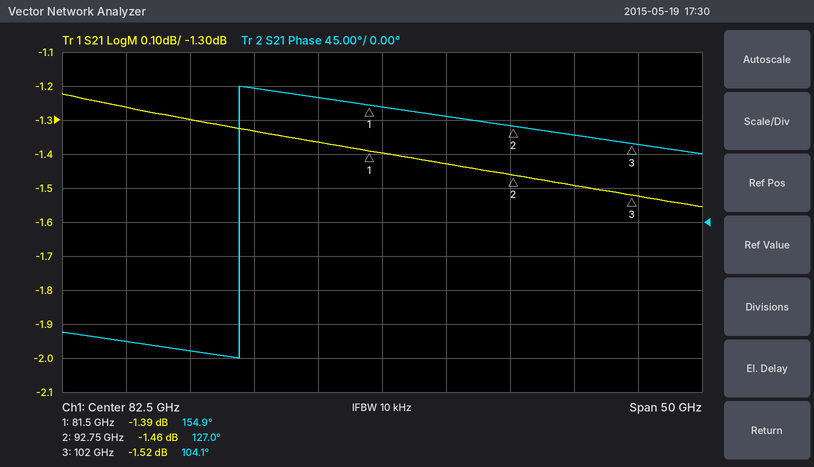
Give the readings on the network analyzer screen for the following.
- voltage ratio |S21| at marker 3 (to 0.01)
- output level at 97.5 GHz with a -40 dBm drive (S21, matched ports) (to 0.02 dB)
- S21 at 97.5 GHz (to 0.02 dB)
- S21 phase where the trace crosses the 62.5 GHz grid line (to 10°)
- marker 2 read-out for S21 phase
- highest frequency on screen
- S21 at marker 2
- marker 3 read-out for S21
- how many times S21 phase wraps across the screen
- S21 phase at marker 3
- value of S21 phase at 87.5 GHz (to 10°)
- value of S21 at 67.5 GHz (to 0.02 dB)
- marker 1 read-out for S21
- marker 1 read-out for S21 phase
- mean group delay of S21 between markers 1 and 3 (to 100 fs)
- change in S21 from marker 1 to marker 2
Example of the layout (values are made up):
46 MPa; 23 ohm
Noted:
0.84; -41.50 dBm; -1.50 dB; -160°; 127.0°; 107.5 GHz; -1.46 dB; -1.52 dB; 1; 104.1°; 140°; -1.30 dB; -1.39 dB; 154.9°; 6.9 ps; -0.07 dB
